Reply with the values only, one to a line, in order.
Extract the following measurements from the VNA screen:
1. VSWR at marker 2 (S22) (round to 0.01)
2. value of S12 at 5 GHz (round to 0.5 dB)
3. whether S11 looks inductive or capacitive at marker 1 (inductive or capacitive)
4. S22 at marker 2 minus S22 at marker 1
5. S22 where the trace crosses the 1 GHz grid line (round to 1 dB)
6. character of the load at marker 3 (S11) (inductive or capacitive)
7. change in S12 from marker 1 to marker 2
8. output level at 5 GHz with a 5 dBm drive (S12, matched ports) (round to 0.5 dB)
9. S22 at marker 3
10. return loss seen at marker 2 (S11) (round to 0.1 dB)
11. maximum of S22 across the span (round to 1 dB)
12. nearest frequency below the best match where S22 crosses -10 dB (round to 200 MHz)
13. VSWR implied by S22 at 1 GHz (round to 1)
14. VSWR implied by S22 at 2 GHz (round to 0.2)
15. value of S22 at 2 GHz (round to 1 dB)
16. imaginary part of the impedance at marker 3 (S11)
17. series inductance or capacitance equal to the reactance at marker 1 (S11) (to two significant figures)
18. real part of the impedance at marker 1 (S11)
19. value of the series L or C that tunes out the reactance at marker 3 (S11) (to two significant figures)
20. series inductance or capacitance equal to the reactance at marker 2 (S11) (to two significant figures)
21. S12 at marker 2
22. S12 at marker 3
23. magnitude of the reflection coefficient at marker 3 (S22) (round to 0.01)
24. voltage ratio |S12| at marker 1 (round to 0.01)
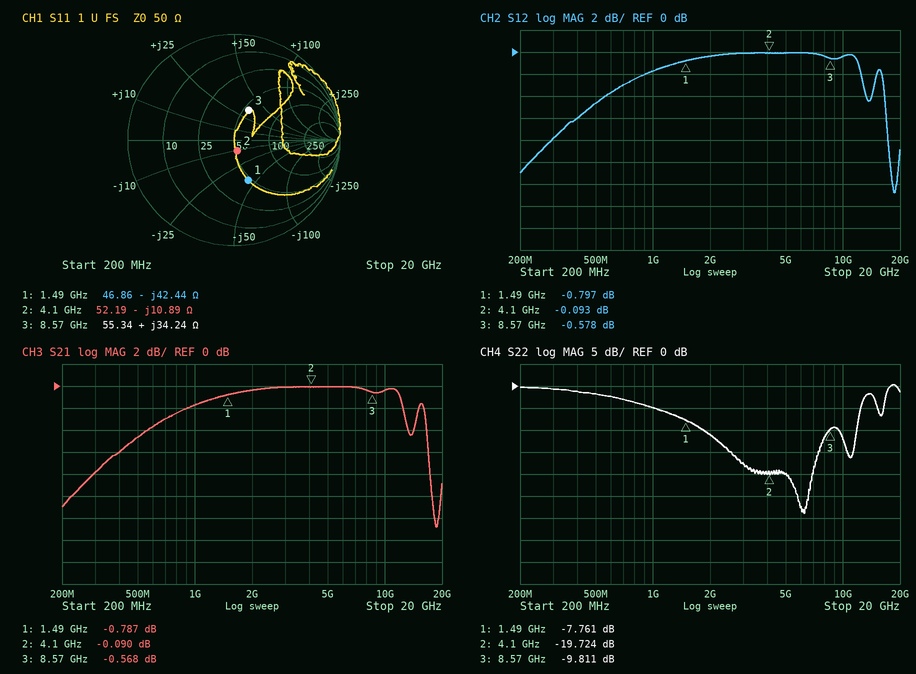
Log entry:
1.23
0.0 dB
capacitive
-11.963 dB
-5 dB
inductive
0.704 dB
5.0 dBm
-9.811 dB
19.3 dB
0 dB
1.8 GHz
4
1.8
-11 dB
+34.24 Ω
2.5 pF
46.86 Ω
540 fF
3.6 pF
-0.093 dB
-0.578 dB
0.32
0.91
